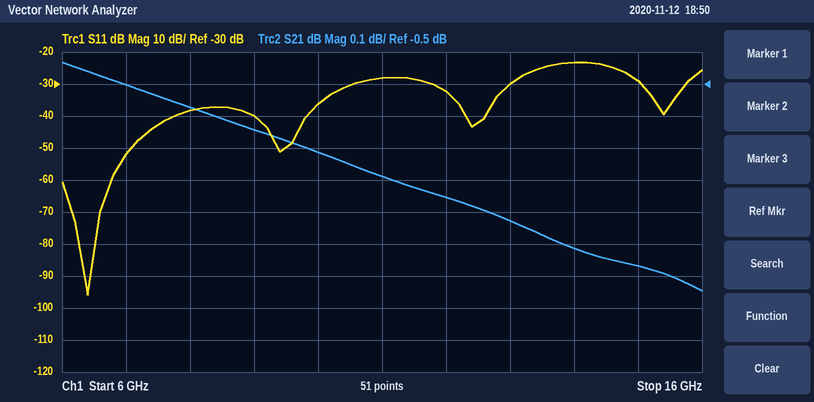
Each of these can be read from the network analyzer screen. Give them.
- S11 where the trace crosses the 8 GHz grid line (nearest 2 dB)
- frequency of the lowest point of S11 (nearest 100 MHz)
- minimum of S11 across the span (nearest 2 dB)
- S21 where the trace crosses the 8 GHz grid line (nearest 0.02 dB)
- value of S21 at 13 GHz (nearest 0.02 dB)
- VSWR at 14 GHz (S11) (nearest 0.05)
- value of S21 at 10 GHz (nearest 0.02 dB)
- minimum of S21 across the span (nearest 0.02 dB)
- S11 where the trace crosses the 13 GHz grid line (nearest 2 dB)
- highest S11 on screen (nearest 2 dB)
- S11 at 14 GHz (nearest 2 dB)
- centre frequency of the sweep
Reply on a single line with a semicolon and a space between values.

-38 dB; 6.4 GHz; -96 dB; -0.58 dB; -0.92 dB; 1.15; -0.72 dB; -1.14 dB; -30 dB; -24 dB; -24 dB; 11 GHz
